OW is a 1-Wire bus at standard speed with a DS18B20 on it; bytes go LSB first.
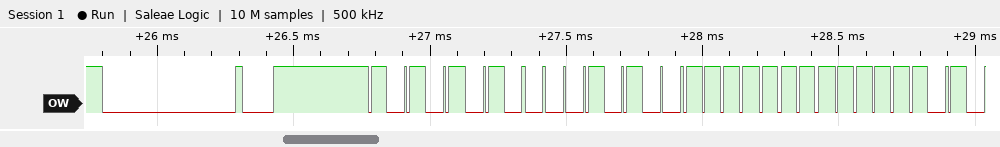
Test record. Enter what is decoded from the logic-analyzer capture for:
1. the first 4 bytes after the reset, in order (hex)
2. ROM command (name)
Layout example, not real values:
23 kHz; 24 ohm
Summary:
55 28 FF 5F; Match ROM
